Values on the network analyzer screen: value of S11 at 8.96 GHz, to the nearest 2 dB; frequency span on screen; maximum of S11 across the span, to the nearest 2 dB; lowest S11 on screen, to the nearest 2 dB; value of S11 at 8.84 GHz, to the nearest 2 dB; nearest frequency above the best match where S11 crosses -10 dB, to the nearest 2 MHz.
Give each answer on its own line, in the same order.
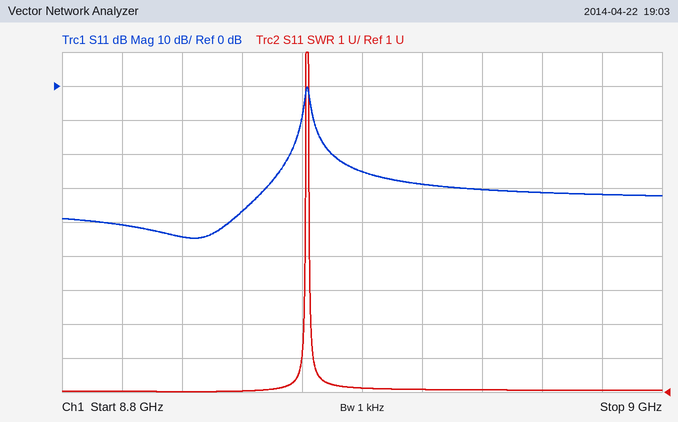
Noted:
-32 dB
200 MHz
0 dB
-44 dB
-44 dB
8.880 GHz
